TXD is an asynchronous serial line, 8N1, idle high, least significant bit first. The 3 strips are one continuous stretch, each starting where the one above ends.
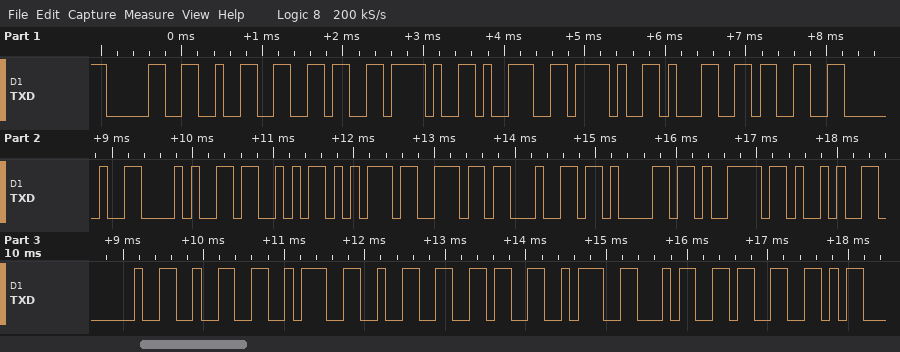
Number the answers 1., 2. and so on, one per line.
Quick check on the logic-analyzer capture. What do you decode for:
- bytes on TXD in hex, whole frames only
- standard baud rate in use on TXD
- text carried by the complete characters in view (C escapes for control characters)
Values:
1. 30 32 36 2F 39 2F 31 33 20 28 53 75 6E 64 61 79 29 20 32 3A 32 36 3A 34 33
2. 9600 baud
3. "026/9/13 (Sunday) 2:26:43"
